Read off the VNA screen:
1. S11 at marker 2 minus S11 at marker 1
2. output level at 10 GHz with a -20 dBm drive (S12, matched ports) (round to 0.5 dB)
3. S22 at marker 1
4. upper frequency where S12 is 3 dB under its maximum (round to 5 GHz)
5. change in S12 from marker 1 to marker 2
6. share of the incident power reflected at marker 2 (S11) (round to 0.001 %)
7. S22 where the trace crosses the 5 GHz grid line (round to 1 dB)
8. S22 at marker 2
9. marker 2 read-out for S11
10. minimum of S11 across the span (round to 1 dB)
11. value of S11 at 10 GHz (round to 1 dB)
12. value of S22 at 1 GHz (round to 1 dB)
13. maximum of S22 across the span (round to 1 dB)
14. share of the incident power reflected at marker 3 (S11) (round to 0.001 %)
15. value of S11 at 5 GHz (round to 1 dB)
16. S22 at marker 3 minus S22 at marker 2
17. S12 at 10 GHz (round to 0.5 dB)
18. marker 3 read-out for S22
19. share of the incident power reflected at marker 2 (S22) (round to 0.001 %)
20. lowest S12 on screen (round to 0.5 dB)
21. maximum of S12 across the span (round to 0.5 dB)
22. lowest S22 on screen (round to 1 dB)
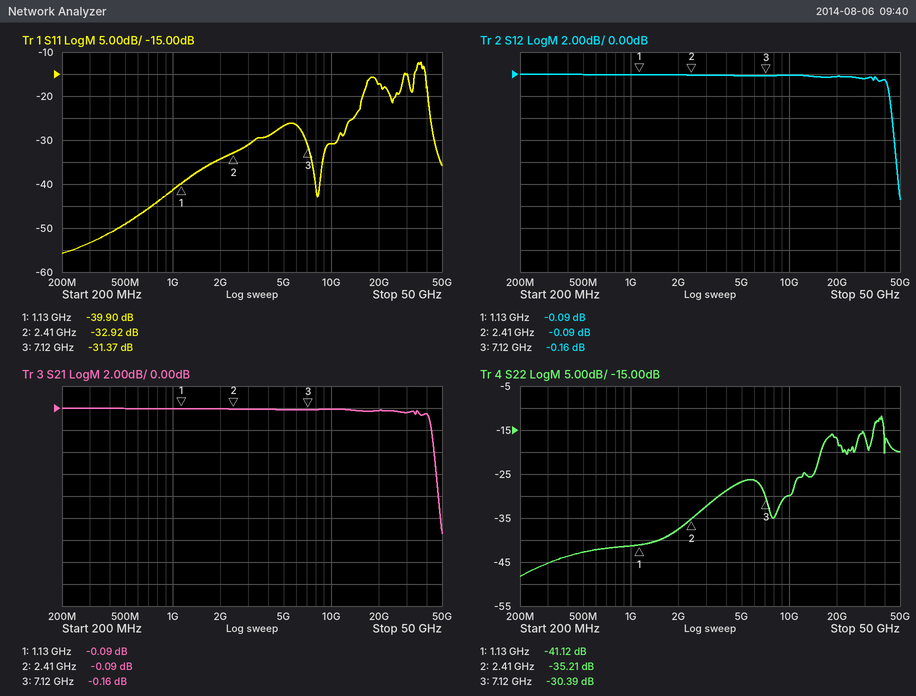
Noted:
6.98 dB
-20.0 dBm
-41.12 dB
45 GHz
0.00 dB
0.051 %
-27 dB
-35.21 dB
-32.92 dB
-56 dB
-31 dB
-41 dB
-12 dB
0.073 %
-27 dB
4.82 dB
0.0 dB
-30.39 dB
0.030 %
-11.5 dB
0.0 dB
-48 dB
